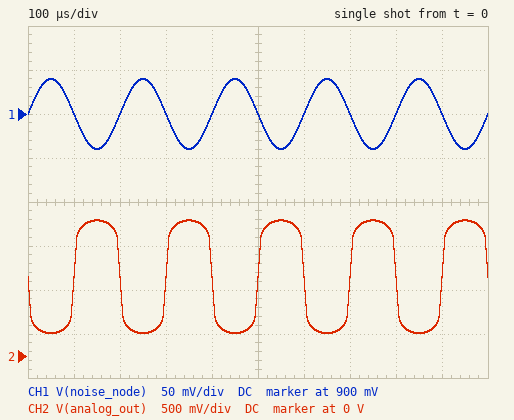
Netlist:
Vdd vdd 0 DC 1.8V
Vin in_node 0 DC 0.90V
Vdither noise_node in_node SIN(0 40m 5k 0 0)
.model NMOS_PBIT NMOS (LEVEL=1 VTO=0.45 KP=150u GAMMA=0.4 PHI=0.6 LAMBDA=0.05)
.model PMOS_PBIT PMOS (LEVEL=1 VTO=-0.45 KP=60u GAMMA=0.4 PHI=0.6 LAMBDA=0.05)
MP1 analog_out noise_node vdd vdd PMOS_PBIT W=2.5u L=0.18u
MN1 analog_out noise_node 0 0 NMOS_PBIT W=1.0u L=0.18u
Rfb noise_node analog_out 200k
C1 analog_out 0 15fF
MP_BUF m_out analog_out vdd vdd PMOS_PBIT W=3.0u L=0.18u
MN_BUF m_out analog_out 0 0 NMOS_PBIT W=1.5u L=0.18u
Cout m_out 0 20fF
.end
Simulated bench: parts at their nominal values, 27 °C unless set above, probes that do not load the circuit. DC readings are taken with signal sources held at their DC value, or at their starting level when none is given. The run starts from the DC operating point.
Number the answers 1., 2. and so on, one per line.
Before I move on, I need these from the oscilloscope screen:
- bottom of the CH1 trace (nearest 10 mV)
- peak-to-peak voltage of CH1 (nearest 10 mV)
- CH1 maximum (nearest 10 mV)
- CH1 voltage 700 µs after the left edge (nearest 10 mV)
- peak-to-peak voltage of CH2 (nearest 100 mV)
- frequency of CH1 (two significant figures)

1. 860 mV
2. 80 mV
3. 940 mV
4. 900 mV
5. 1.3 V
6. 5.0 kHz
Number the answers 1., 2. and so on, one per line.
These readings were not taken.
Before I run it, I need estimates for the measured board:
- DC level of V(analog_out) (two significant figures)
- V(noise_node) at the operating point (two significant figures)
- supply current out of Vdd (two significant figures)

1. 900 mV
2. 900 mV
3. 200 µA
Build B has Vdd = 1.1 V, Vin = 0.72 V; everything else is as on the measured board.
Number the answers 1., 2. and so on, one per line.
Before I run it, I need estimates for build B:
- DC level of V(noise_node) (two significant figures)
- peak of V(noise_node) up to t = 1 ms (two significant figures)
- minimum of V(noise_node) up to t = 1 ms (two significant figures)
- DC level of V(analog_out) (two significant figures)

1. 720 mV
2. 760 mV
3. 680 mV
4. 16 mV
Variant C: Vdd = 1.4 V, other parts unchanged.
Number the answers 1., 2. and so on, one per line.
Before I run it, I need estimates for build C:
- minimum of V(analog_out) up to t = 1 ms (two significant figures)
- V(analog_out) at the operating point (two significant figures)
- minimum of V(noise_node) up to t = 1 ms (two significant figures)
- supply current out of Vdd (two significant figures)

1. 12 mV
2. 15 mV
3. 860 mV
4. 1.1 µA
